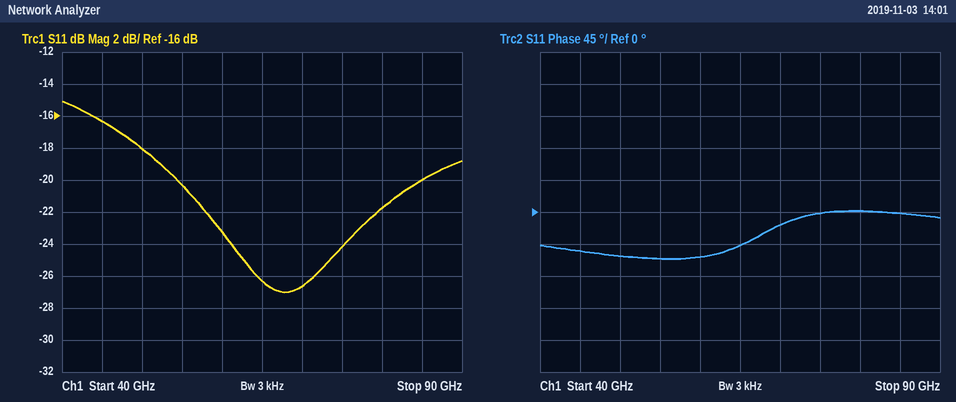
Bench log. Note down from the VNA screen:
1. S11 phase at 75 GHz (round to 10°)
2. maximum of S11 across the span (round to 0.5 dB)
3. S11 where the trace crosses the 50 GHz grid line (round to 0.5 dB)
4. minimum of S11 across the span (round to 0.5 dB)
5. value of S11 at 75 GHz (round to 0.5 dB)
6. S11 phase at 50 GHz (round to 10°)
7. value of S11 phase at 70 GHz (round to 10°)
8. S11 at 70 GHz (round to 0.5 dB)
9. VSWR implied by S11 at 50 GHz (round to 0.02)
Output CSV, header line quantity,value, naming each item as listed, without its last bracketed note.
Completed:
quantity,value
S11 phase at 75 GHz,0°
maximum of S11 across the span,-15.0 dB
S11 where the trace crosses the 50 GHz grid line,-18.0 dB
minimum of S11 across the span,-27.0 dB
value of S11 at 75 GHz,-24.0 dB
S11 phase at 50 GHz,-60°
value of S11 phase at 70 GHz,-20°
S11 at 70 GHz,-26.5 dB
VSWR implied by S11 at 50 GHz,1.28
